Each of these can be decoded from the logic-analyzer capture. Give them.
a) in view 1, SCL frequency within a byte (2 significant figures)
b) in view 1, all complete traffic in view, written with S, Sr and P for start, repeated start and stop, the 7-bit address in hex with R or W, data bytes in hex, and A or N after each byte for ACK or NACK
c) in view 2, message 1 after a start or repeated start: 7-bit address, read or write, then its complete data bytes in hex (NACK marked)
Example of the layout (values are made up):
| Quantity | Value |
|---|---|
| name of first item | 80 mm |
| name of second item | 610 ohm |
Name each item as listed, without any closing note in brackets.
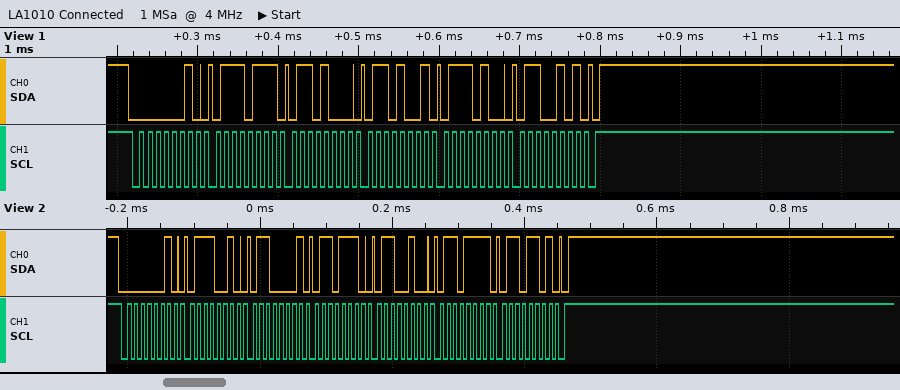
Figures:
| Quantity | Value |
|---|---|
| in view 1, SCL frequency within a byte | 100 kHz |
| in view 1, all complete traffic in view, written with S, Sr and P for start, repeated start and stop, the 7-bit address in hex with R or W, data bytes in hex, and A or N after each byte for ACK or NACK | S 01W A 77 A 68 A 69 A 74 A 65 A P |
| in view 2, message 1 after a start or repeated start: 7-bit address, read or write, then its complete data bytes in hex | 0x01 write: 72 61 6E 64 6F 6D |
